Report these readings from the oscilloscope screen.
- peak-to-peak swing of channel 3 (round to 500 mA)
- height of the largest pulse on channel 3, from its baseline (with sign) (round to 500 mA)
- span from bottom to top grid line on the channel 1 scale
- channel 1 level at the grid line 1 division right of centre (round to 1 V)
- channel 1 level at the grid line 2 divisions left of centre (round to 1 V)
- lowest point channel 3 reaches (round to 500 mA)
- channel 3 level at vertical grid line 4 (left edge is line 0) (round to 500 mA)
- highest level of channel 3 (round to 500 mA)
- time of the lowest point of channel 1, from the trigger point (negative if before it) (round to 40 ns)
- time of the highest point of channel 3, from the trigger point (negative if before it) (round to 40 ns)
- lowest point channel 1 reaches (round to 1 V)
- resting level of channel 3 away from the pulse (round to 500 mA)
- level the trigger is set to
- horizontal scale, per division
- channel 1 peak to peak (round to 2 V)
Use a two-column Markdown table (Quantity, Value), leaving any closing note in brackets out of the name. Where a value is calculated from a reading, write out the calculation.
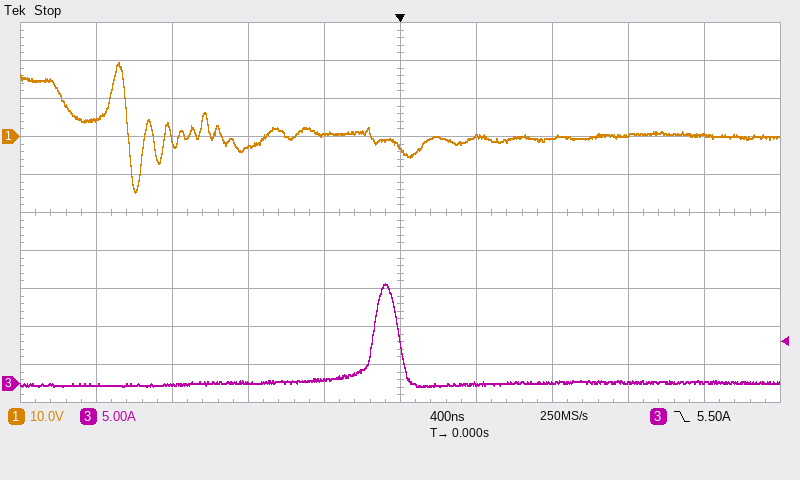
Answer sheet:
| Quantity | Value |
|---|---|
| peak-to-peak swing of channel 3 | 13.0 A − (-500 mA) = 13.5 A |
| height of the largest pulse on channel 3, from its baseline (with sign) | 13.0 A − (0.0 A) = +13.0 A |
| span from bottom to top grid line on the channel 1 scale | 100 V |
| channel 1 level at the grid line 1 division right of centre | 0 V |
| channel 1 level at the grid line 2 divisions left of centre | -3 V |
| lowest point channel 3 reaches | -500 mA |
| channel 3 level at vertical grid line 4 (left edge is line 0) | 500 mA |
| highest level of channel 3 | 13.0 A |
| time of the lowest point of channel 1, from the trigger point (negative if before it) | -1.40 µs |
| time of the highest point of channel 3, from the trigger point (negative if before it) | -80 ns |
| lowest point channel 1 reaches | -15 V |
| resting level of channel 3 away from the pulse | 0.0 A |
| level the trigger is set to | 5.50 A |
| horizontal scale, per division | 400 ns |
| channel 1 peak to peak | 34 V |
